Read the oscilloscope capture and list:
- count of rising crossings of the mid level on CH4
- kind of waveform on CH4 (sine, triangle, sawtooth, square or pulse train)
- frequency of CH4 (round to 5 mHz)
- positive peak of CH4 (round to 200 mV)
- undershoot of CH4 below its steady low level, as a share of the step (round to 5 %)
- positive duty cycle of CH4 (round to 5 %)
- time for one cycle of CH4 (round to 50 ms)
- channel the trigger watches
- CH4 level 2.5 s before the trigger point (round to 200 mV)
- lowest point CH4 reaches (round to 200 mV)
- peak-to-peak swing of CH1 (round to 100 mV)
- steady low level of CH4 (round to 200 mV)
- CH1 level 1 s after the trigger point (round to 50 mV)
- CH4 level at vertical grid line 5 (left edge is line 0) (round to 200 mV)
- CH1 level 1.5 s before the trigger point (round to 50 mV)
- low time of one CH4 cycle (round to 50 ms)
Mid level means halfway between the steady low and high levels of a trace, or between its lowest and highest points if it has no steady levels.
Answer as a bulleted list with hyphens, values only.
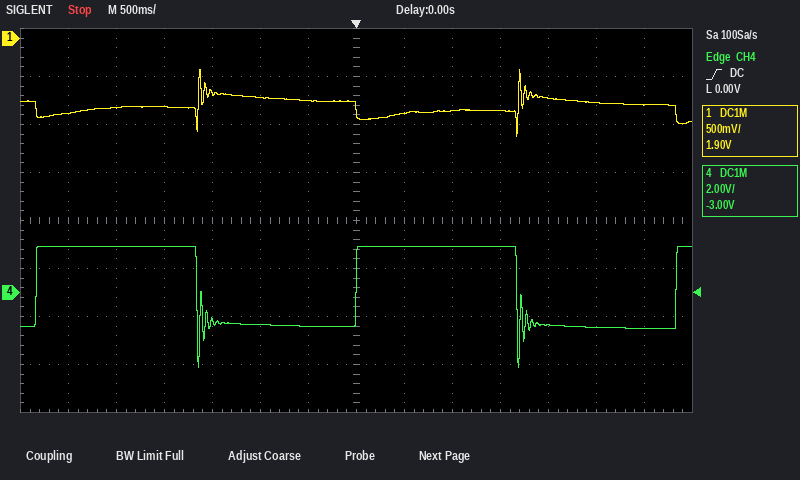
- 3
- square
- 300 mHz
- 2.0 V
- 50 %
- 50 %
- 3.35 s
- CH4
- 2.0 V
- -3.2 V
- 700 mV
- -1.4 V
- -750 mV
- -1.4 V
- -550 mV
- 1.65 s
